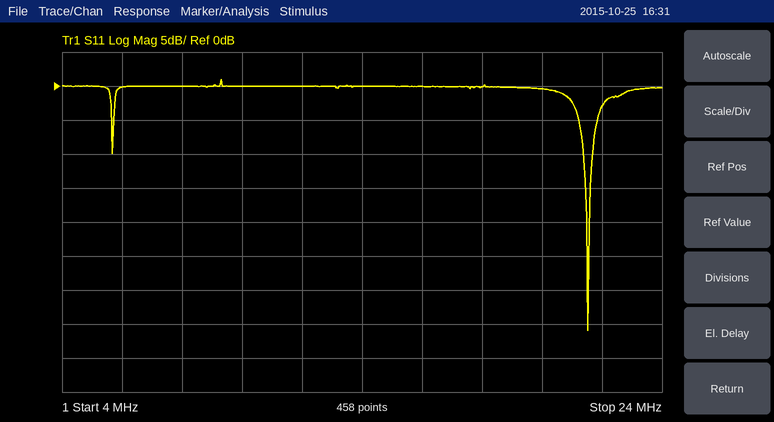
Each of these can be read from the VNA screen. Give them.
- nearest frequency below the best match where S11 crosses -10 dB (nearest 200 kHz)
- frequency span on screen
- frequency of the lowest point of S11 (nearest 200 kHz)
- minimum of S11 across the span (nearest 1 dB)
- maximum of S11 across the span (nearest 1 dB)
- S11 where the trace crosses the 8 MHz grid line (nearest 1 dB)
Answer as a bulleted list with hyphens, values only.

- 21.4 MHz
- 20 MHz
- 21.6 MHz
- -36 dB
- 1 dB
- 0 dB
